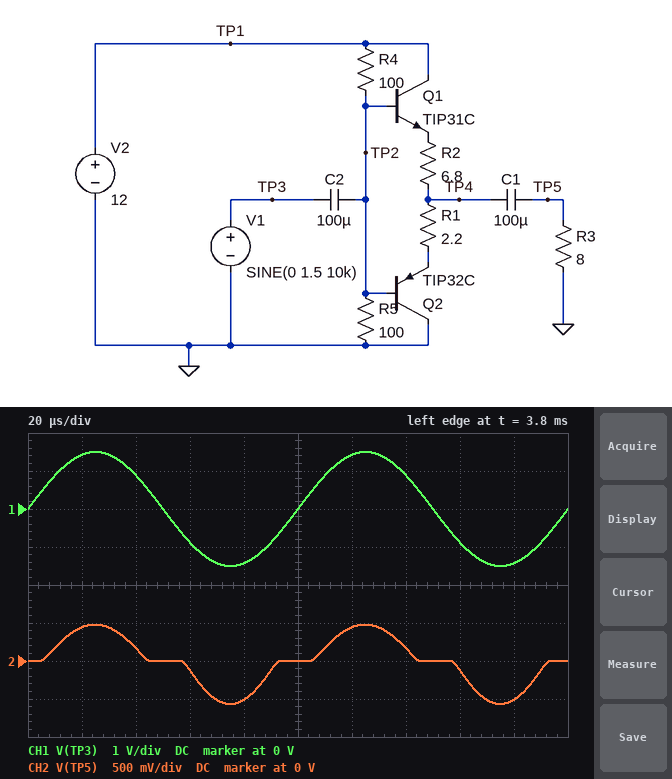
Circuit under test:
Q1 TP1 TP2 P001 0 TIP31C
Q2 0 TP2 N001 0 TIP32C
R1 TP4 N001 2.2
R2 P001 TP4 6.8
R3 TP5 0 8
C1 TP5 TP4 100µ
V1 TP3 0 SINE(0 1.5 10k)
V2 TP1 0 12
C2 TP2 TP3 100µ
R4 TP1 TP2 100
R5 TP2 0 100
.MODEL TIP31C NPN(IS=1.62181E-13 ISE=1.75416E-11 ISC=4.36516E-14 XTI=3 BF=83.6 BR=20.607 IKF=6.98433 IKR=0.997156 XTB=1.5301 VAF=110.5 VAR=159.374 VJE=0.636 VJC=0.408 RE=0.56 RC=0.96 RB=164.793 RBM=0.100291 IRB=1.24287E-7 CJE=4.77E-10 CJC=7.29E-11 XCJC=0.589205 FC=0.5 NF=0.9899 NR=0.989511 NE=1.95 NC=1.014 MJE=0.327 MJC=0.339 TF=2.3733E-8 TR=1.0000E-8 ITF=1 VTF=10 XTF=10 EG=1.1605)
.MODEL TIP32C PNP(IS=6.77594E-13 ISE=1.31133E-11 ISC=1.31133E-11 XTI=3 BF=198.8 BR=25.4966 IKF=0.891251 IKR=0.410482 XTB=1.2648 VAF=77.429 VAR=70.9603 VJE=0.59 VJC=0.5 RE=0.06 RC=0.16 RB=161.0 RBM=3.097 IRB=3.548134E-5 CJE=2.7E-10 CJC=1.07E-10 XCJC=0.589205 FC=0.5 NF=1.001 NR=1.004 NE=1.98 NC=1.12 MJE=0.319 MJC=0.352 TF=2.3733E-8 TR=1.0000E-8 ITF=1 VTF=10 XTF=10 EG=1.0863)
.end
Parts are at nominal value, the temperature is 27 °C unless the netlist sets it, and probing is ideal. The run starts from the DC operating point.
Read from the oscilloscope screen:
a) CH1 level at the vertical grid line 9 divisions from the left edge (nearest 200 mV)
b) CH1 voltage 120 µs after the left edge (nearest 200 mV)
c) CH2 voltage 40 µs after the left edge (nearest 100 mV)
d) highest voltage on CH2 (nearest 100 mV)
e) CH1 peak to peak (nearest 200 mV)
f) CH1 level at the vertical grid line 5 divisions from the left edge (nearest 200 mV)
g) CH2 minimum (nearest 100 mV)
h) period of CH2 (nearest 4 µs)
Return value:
-1.4 V
1.4 V
200 mV
500 mV
3.0 V
0 V
-600 mV
100 µs
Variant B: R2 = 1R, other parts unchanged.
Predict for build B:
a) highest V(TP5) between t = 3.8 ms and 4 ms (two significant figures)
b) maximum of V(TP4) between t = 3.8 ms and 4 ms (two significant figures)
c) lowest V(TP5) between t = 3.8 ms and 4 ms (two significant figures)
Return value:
670 mV
6.7 V
-650 mV
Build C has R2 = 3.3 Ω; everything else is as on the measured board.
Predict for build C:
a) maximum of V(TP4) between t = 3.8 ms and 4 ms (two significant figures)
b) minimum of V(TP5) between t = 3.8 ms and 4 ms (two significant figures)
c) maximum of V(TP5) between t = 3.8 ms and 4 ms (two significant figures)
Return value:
6.5 V
-610 mV
580 mV
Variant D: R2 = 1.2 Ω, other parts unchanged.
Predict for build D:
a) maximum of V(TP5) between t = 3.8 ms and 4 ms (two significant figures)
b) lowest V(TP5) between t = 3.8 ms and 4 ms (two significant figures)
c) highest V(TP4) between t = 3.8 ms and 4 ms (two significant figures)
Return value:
660 mV
-650 mV
6.7 V
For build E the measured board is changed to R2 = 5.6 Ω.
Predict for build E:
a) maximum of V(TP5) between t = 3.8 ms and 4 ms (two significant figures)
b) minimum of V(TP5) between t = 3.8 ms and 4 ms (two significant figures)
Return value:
510 mV
-580 mV
